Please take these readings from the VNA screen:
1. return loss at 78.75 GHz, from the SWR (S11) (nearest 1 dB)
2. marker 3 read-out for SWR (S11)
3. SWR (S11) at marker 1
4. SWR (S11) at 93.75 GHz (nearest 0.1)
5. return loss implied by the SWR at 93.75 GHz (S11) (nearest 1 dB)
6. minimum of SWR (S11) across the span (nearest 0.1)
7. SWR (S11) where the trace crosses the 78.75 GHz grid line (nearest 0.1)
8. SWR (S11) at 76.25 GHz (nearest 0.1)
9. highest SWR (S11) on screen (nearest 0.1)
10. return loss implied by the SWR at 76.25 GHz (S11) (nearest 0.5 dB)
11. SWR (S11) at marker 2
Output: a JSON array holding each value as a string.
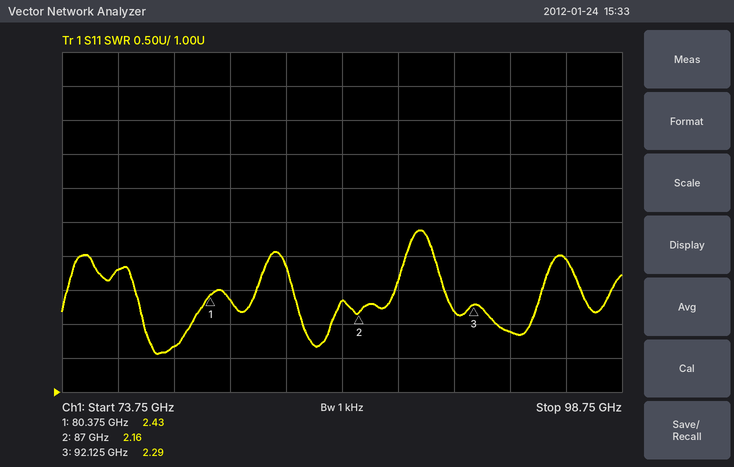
["12 dB", "2.29", "2.43", "1.9", "10 dB", "1.6", "1.7", "2.8", "3.4", "6.5 dB", "2.16"]
